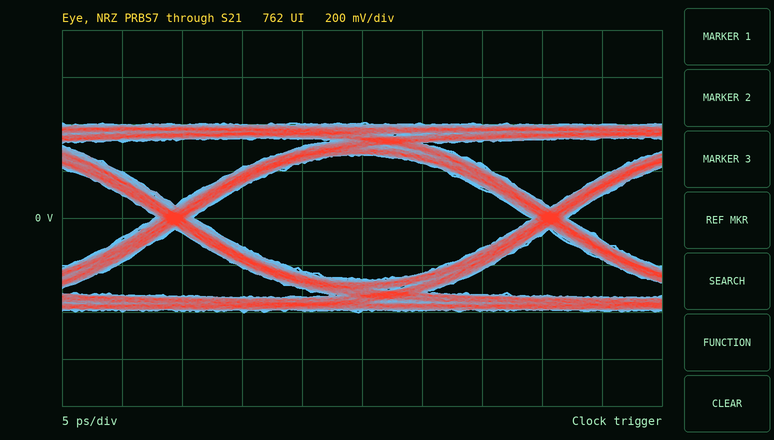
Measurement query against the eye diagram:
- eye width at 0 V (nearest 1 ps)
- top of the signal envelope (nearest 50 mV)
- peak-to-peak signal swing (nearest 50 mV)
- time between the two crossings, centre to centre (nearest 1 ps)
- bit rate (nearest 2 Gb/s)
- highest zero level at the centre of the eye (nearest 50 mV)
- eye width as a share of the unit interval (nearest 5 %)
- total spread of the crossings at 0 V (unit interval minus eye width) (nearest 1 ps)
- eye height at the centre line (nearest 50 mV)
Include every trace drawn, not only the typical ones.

28 ps
400 mV
800 mV
31 ps
32 Gb/s
-250 mV
90 %
3 ps
550 mV
